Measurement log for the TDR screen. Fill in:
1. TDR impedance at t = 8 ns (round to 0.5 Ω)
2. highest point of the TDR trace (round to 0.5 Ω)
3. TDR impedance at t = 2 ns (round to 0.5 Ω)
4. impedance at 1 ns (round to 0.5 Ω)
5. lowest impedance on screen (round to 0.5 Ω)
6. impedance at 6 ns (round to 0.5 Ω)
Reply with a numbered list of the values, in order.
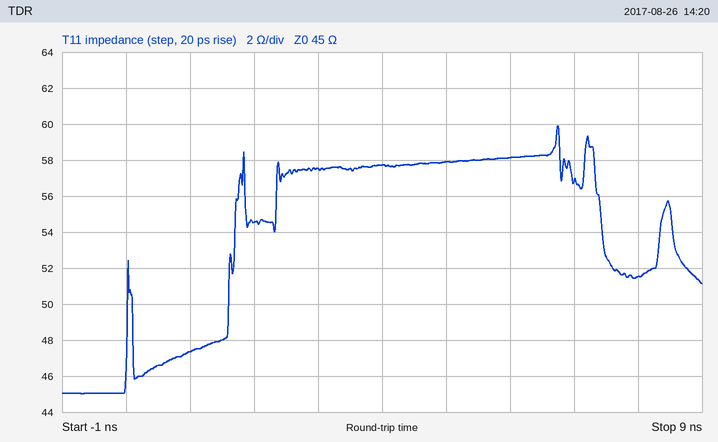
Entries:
1. 51.5 Ω
2. 60.0 Ω
3. 54.5 Ω
4. 47.5 Ω
5. 45.0 Ω
6. 58.0 Ω
